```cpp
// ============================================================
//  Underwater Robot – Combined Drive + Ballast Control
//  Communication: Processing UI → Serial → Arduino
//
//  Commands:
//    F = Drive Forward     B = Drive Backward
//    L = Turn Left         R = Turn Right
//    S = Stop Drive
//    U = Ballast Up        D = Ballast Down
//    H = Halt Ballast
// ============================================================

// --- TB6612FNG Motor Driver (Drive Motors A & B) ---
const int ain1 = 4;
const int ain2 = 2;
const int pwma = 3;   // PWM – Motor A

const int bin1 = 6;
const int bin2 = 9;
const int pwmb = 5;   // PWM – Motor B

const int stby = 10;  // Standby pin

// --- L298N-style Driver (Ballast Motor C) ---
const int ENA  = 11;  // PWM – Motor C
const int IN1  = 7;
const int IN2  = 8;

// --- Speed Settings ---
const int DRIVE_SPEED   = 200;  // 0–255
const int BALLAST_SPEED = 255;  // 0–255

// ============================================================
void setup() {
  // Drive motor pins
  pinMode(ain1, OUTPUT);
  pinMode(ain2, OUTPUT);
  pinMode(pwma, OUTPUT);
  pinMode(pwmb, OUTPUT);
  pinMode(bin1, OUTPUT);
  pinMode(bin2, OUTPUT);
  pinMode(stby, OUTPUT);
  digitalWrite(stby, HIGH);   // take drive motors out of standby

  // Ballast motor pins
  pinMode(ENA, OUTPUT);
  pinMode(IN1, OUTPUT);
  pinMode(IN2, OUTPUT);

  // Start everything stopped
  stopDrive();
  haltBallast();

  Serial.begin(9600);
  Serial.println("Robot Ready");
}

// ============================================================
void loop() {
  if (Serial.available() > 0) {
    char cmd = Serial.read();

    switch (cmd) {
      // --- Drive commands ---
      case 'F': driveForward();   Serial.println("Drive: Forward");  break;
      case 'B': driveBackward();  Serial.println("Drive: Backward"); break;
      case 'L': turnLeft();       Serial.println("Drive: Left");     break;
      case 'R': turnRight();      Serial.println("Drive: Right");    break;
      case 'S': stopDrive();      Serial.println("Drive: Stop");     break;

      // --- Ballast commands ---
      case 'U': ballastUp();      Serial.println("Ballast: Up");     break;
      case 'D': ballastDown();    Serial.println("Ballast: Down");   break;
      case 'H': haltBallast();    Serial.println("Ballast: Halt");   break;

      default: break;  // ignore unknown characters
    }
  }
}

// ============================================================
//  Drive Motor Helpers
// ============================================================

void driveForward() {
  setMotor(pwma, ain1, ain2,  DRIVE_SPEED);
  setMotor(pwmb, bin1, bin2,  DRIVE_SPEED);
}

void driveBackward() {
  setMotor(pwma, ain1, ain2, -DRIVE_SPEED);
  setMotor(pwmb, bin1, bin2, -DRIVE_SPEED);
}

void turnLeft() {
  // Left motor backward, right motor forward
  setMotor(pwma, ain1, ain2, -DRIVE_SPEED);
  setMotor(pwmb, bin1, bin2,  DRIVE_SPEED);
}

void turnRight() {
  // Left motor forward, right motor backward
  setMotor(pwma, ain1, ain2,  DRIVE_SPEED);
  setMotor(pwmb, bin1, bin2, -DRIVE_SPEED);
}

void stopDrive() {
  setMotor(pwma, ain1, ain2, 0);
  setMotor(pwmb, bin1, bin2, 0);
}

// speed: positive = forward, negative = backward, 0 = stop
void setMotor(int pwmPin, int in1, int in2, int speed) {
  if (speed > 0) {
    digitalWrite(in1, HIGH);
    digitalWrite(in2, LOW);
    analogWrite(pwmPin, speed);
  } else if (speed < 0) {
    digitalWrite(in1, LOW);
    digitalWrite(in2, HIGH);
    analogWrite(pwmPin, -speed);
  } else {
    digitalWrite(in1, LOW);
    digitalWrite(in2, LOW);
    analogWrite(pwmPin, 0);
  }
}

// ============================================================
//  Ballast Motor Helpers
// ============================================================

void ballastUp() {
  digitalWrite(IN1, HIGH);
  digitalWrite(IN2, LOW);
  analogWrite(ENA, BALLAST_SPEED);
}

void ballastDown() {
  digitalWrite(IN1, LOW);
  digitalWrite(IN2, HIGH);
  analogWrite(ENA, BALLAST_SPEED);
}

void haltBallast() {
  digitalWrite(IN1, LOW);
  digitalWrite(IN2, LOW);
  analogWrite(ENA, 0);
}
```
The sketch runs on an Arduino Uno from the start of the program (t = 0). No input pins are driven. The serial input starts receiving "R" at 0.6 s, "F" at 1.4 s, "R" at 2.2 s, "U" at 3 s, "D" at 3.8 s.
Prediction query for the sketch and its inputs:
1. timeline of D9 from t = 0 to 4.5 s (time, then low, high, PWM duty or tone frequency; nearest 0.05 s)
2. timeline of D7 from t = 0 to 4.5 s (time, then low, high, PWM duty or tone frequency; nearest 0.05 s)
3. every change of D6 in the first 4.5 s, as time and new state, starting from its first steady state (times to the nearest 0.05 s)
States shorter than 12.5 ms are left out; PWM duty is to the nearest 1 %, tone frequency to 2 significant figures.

0 s low; 0.6 s high; 1.4 s low; 2.2 s high
0 s low; 3 s high; 3.8 s low
0 s low; 1.4 s high; 2.2 s low
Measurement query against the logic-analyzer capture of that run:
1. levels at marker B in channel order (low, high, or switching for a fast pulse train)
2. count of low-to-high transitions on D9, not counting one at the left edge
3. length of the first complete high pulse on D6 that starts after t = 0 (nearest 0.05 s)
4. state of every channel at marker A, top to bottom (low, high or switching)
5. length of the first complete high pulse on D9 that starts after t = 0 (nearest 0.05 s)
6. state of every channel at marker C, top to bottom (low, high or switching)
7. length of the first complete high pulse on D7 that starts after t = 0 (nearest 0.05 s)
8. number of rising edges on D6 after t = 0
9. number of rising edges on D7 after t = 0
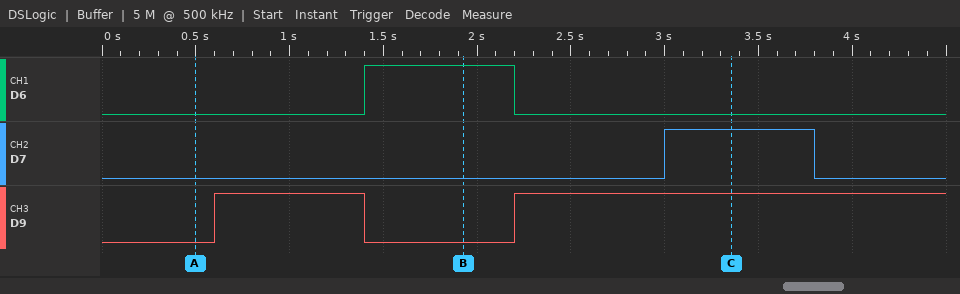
D6 high, D7 low, D9 low
2
0.80 s
D6 low, D7 low, D9 low
0.80 s
D6 low, D7 high, D9 high
0.80 s
1
1
